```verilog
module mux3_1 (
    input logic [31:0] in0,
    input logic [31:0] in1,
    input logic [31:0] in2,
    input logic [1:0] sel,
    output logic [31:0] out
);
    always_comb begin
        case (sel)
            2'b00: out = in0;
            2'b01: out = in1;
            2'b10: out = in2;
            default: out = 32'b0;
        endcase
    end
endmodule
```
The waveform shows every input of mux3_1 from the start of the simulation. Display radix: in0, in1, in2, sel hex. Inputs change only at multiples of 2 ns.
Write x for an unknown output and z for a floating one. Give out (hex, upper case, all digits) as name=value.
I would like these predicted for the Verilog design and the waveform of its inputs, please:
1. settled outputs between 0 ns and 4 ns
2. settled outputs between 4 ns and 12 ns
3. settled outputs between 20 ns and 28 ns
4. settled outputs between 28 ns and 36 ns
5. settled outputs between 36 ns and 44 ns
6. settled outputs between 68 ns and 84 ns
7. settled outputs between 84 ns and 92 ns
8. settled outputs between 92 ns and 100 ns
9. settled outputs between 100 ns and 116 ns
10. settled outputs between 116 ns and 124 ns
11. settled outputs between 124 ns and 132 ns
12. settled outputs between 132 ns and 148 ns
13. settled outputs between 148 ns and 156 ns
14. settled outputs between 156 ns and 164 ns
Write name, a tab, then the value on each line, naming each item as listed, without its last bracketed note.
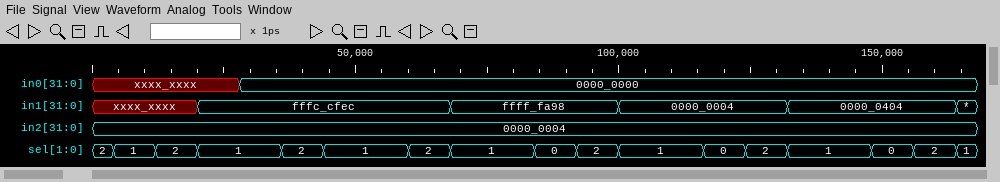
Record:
settled outputs between 0 ns and 4 ns	out=00000004
settled outputs between 4 ns and 12 ns	out=x
settled outputs between 20 ns and 28 ns	out=FFFCCFEC
settled outputs between 28 ns and 36 ns	out=FFFCCFEC
settled outputs between 36 ns and 44 ns	out=00000004
settled outputs between 68 ns and 84 ns	out=FFFFFA98
settled outputs between 84 ns and 92 ns	out=00000000
settled outputs between 92 ns and 100 ns	out=00000004
settled outputs between 100 ns and 116 ns	out=00000004
settled outputs between 116 ns and 124 ns	out=00000000
settled outputs between 124 ns and 132 ns	out=00000004
settled outputs between 132 ns and 148 ns	out=00000404
settled outputs between 148 ns and 156 ns	out=00000000
settled outputs between 156 ns and 164 ns	out=00000004
